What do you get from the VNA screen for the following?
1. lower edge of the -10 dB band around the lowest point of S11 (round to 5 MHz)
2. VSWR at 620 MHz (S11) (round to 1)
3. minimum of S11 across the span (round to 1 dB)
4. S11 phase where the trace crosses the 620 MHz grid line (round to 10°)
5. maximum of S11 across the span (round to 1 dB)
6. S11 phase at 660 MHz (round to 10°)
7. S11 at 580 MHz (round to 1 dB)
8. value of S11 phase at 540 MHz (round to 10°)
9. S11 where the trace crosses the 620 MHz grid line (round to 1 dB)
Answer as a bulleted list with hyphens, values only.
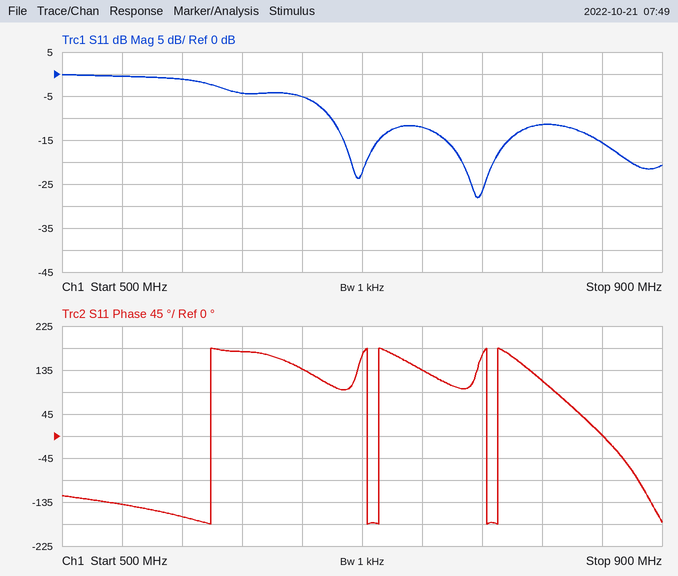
- 680 MHz
- 4
- -28 dB
- 170°
- 0 dB
- 140°
- -1 dB
- -140°
- -4 dB
